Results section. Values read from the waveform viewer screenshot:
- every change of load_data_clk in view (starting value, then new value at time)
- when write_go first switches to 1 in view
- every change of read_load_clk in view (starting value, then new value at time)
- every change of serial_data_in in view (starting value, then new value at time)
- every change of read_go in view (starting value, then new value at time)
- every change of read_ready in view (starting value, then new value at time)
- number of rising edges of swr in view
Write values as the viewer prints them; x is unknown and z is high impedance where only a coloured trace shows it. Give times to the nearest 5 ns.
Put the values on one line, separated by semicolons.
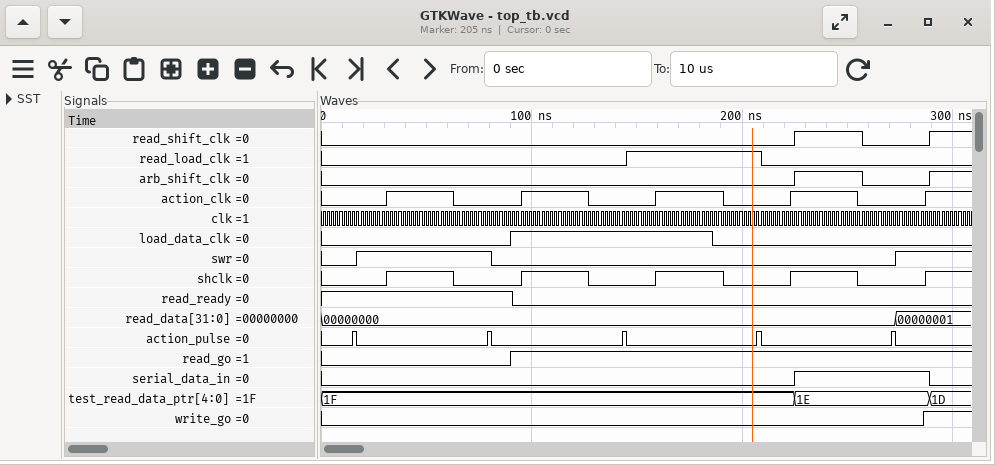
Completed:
0, 1 at 90 ns, 0 at 185 ns; 285 ns; 0, 1 at 145 ns, 0 at 210 ns; 0, 1 at 225 ns, 0 at 290 ns; 0, 1 at 90 ns; 1, 0 at 90 ns; 2
